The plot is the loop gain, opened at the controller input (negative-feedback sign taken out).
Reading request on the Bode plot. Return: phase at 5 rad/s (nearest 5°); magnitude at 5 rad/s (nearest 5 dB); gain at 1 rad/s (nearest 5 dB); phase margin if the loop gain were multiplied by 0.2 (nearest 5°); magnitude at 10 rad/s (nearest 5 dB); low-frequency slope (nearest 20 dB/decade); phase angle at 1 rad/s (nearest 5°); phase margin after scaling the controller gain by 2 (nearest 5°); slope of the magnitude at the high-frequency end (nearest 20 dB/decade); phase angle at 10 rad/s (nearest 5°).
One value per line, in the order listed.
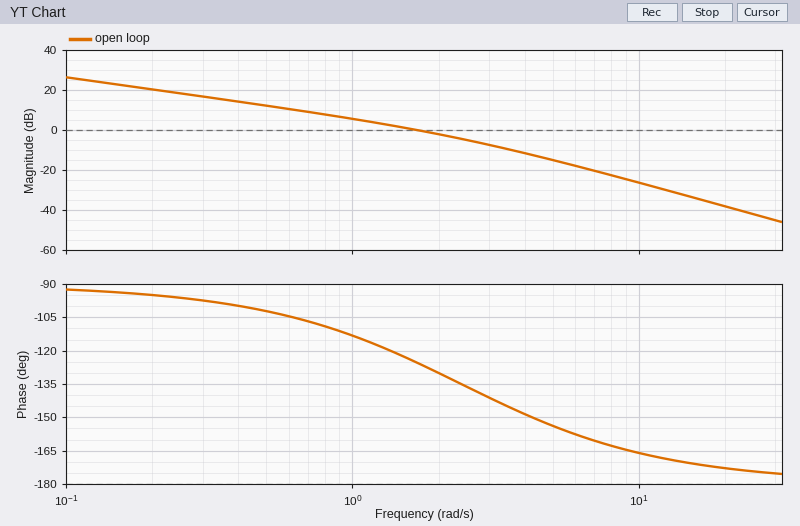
-155°
-15 dB
5 dB
80°
-25 dB
-20 dB/decade
-115°
40°
-40 dB/decade
-165°
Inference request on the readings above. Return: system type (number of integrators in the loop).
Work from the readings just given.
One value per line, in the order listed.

1
